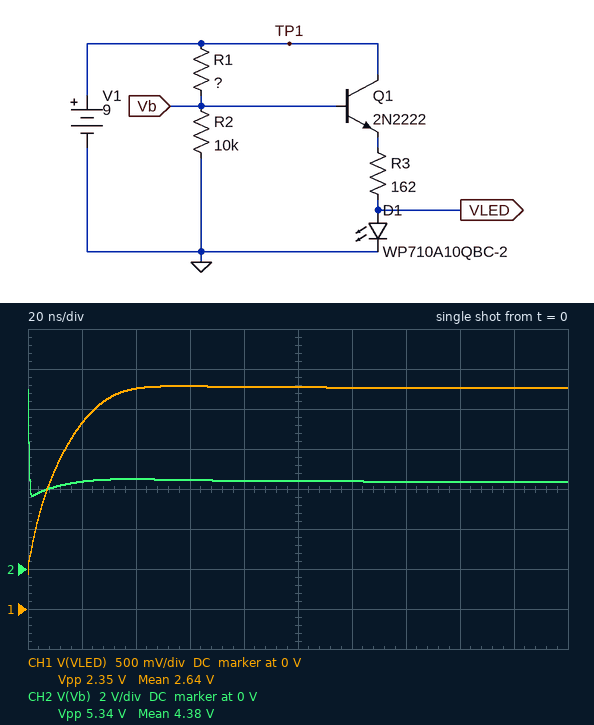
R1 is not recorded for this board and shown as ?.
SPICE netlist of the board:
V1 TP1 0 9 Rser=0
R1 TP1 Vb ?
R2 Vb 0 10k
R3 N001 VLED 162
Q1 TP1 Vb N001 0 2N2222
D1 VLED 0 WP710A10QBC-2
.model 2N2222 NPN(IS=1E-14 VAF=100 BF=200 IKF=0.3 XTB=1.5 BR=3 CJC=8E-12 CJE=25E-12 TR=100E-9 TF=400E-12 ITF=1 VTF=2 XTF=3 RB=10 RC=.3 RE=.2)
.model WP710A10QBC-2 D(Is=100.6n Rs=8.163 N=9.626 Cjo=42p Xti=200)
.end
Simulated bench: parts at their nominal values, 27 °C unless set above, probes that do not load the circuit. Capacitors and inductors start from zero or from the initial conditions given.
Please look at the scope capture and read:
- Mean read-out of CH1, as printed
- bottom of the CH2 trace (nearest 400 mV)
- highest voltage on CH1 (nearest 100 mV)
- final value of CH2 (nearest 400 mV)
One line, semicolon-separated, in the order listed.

2.64 V; 3.6 V; 2.8 V; 4.4 V
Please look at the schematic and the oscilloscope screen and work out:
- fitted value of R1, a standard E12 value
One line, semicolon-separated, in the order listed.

10 kΩ
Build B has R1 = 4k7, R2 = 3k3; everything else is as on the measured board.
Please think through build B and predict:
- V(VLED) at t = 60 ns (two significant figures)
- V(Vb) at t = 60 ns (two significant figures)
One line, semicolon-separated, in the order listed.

2.6 V; 3.7 V
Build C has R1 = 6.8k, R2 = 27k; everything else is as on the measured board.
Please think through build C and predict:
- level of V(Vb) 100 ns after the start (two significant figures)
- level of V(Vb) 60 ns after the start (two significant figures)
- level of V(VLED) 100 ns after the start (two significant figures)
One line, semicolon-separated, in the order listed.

6.6 V; 6.4 V; 3.1 V
